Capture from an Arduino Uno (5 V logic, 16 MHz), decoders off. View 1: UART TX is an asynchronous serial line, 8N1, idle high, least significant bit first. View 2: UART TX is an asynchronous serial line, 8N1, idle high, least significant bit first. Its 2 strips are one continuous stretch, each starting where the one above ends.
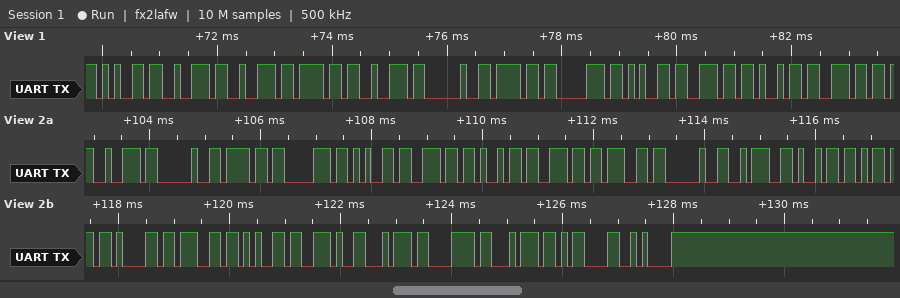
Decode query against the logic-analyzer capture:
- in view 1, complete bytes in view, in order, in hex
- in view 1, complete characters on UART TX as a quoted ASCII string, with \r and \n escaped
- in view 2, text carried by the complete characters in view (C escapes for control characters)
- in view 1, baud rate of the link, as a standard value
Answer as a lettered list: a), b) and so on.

a) 65 72 72 6F 72 20 6F 70 65 6E 69 6E
b) "error openin"
c) "r opening :image.txt\r\n"
d) 9600 baud
